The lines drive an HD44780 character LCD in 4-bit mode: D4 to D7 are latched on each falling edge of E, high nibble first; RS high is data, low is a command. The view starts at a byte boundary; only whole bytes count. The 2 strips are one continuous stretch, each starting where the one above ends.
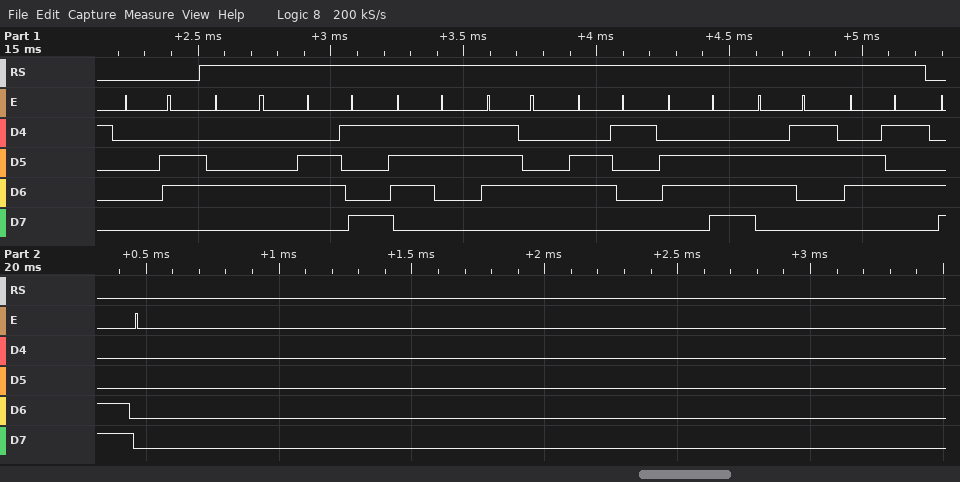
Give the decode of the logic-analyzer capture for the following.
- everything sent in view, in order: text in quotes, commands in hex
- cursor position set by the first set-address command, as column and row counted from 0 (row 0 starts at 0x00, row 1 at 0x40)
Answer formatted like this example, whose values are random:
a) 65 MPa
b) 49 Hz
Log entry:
a) 0x06 "Distance" 0xC0
b) column 0, row 1
